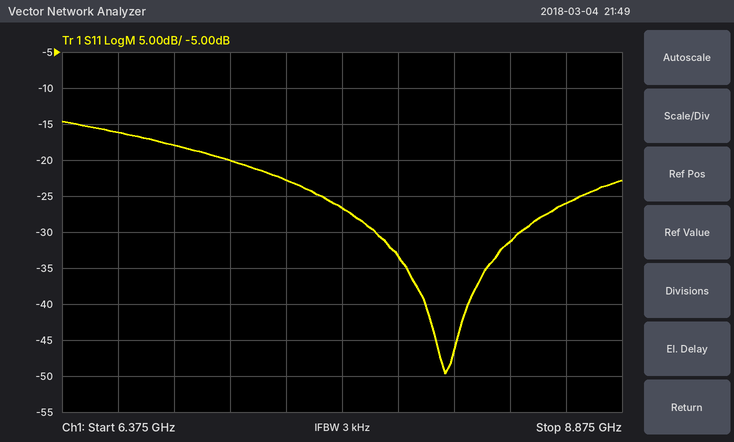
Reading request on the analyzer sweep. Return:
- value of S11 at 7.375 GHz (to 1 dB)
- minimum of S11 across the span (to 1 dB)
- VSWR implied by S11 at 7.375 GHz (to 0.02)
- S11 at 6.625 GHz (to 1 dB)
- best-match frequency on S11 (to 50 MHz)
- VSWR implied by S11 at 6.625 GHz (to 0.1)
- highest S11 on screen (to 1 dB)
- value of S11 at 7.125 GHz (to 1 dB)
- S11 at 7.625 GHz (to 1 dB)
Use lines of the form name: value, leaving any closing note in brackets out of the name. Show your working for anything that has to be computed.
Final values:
value of S11 at 7.375 GHz: -23 dB
minimum of S11 across the span: -50 dB
VSWR implied by S11 at 7.375 GHz: |Γ| = 10^(-23/20) = 0.0708; VSWR = (1 + 0.0708)/(1 − 0.0708) ≈ 1.15, so 1.16 to the nearest 0.02
S11 at 6.625 GHz: -16 dB
best-match frequency on S11: 8.10 GHz
VSWR implied by S11 at 6.625 GHz: |Γ| = 10^(-16/20) = 0.1585; VSWR = (1 + 0.1585)/(1 − 0.1585) ≈ 1.4
highest S11 on screen: -15 dB
value of S11 at 7.125 GHz: -20 dB
S11 at 7.625 GHz: -27 dB
